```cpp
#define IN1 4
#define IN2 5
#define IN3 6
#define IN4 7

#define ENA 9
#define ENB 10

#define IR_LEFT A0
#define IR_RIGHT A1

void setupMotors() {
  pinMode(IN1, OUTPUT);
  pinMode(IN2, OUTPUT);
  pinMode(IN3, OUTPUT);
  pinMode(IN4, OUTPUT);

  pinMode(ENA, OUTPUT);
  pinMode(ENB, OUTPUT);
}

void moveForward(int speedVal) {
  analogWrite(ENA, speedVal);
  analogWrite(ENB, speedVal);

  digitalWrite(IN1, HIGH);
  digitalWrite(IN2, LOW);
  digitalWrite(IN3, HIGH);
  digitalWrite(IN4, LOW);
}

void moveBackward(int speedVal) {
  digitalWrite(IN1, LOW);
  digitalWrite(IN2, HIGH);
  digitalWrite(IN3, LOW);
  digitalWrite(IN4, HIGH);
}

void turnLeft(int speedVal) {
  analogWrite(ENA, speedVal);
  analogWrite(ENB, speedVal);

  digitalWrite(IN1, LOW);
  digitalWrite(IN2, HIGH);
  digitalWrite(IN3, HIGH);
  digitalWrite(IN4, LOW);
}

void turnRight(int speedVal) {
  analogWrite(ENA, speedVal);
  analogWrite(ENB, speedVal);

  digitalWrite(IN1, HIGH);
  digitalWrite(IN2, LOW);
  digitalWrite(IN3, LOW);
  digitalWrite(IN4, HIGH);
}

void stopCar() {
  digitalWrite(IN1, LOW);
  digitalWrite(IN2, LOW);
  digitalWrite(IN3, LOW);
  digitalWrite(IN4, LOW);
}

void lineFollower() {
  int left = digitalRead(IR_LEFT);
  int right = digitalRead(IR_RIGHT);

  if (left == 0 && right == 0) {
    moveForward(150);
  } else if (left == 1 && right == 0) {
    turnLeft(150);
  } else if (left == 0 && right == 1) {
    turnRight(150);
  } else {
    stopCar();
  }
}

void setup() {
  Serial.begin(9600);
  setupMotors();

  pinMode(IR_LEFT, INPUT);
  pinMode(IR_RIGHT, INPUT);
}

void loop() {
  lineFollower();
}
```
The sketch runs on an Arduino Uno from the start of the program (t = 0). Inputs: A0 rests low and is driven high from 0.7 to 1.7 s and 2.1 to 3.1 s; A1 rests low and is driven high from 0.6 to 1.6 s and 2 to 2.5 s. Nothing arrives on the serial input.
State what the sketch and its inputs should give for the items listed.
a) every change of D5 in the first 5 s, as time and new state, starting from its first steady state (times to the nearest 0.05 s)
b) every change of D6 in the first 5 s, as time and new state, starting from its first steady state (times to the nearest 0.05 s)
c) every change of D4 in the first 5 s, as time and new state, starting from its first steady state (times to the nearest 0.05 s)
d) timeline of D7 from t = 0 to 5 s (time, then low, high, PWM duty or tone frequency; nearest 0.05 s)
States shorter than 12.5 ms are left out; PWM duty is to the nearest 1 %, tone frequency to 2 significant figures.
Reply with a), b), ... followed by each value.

a) 0 s low; 1.6 s high; 1.7 s low; 2.5 s high; 3.1 s low
b) 0 s high; 0.6 s low; 1.6 s high; 2 s low; 2.5 s high
c) 0 s high; 0.7 s low; 1.7 s high; 2.1 s low; 3.1 s high
d) 0 s low; 0.6 s high; 0.7 s low; 2 s high; 2.1 s low
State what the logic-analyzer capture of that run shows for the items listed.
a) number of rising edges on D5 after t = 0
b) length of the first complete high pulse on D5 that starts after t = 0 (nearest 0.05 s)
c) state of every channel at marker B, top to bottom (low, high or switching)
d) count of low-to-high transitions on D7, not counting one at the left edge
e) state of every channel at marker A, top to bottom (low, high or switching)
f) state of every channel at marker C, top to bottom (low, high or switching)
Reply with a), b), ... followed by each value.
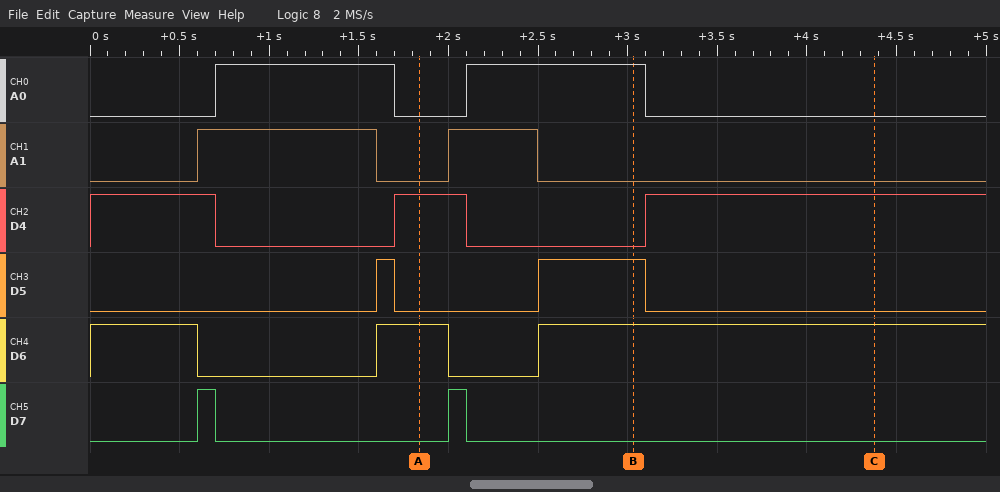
a) 2
b) 0.10 s
c) A0 high, A1 low, D4 low, D5 high, D6 high, D7 low
d) 2
e) A0 low, A1 low, D4 high, D5 low, D6 high, D7 low
f) A0 low, A1 low, D4 high, D5 low, D6 high, D7 low
